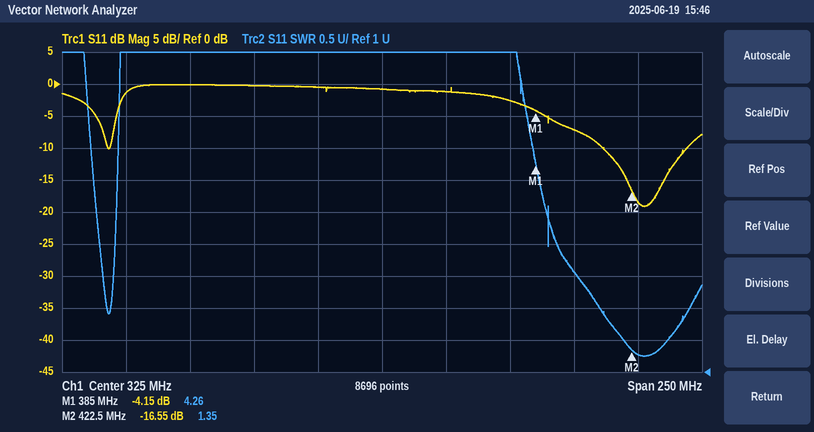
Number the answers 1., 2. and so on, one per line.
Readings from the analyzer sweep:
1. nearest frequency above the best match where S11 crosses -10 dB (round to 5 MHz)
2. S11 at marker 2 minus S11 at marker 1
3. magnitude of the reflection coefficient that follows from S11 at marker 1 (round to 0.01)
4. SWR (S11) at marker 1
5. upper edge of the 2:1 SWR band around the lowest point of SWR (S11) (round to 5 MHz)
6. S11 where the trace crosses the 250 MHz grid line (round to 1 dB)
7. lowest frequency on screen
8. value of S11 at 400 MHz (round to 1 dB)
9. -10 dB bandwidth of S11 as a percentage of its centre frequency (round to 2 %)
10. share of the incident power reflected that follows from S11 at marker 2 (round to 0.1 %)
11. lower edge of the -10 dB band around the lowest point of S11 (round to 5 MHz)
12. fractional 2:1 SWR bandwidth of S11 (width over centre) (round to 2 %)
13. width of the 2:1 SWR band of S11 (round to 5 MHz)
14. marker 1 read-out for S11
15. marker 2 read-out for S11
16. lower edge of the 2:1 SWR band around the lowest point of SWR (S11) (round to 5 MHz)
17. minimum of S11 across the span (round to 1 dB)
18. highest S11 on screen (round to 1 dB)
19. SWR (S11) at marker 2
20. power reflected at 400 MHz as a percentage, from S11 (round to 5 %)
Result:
1. 445 MHz
2. -12.40 dB
3. 0.62
4. 4.26
5. 445 MHz
6. 0 dB
7. 200 MHz
8. -7 dB
9. 8 %
10. 2.2 %
11. 410 MHz
12. 8 %
13. 35 MHz
14. -4.15 dB
15. -16.55 dB
16. 410 MHz
17. -19 dB
18. 0 dB
19. 1.35
20. 20 %
